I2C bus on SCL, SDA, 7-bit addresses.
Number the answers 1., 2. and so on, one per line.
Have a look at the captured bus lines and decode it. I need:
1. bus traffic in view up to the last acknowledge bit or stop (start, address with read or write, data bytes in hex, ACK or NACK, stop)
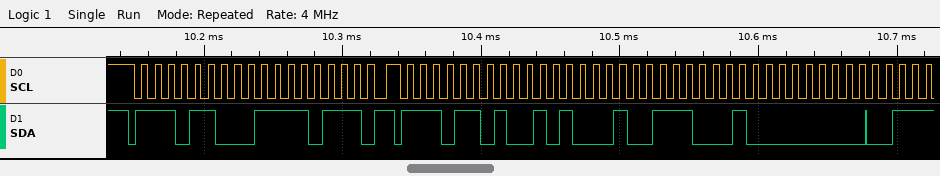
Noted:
1. start, address 76 write ACK, F7 ACK, repeated start, address 76 read ACK, 51 ACK, 71 ACK, 00 ACK
